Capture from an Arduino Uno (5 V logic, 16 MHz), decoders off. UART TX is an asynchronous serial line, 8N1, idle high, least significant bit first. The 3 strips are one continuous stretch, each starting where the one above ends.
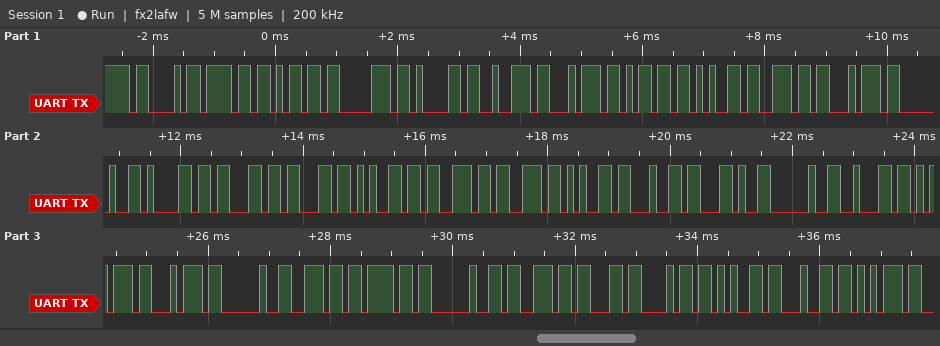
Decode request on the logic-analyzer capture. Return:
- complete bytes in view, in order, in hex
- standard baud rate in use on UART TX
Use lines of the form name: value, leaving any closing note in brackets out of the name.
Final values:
complete bytes in view, in order, in hex: 43 6F 6D 70 61 72 74 6D 65 6E 74 20 61 63 63 65 73 73 65 64 2C 20 62 75 74 20 6E 6F 20 73 63 68 65 64 75
standard baud rate in use on UART TX: 9600 baud
